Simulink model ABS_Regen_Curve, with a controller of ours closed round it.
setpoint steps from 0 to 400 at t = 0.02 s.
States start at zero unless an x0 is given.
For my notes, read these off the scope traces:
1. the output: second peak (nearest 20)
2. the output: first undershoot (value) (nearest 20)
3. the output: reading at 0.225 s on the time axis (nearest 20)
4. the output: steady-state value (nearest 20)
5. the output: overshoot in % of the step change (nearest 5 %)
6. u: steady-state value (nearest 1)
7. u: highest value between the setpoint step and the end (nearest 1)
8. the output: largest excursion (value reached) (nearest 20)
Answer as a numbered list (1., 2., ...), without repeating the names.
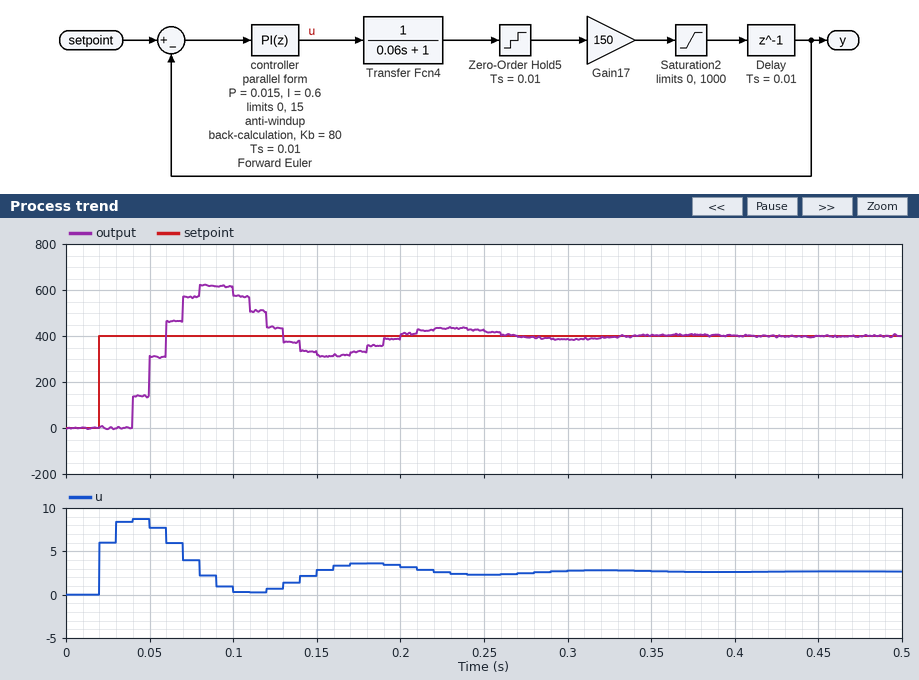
1. 440
2. 320
3. 440
4. 400
5. 55 %
6. 3
7. 9
8. 620
